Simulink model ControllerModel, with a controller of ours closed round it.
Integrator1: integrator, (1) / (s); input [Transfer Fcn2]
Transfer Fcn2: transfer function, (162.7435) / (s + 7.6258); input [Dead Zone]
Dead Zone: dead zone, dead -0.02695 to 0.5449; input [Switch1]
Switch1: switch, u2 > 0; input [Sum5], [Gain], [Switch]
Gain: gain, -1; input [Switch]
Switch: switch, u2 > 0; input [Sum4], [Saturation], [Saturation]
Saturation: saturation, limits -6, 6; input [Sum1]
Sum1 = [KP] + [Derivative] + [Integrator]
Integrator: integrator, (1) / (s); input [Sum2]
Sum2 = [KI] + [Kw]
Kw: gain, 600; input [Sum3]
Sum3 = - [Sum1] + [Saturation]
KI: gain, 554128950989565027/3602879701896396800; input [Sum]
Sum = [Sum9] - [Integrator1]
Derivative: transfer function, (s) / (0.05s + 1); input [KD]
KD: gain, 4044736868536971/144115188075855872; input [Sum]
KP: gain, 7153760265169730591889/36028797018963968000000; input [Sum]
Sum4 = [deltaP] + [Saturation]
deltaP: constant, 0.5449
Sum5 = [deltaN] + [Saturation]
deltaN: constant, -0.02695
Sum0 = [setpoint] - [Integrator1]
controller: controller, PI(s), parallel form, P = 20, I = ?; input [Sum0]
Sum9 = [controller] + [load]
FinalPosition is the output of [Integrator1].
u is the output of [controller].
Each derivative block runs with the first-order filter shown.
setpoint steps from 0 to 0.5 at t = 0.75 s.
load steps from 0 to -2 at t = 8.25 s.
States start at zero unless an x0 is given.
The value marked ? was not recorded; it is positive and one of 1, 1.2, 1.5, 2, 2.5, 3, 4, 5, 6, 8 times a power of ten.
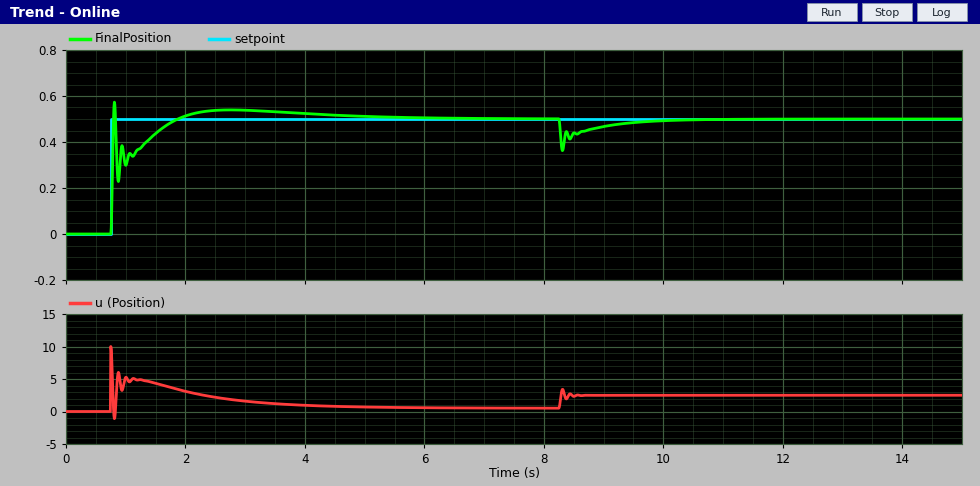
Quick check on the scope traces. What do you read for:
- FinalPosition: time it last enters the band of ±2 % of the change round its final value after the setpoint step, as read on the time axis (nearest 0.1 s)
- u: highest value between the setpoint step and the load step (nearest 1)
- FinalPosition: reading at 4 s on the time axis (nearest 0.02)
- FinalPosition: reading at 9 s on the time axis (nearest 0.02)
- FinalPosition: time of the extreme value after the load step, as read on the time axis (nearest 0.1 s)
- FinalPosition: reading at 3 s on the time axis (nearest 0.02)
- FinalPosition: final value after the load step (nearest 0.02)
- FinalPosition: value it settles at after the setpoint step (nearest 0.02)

5.2 s
10
0.52
0.46
8.3 s
0.54
0.50
0.50
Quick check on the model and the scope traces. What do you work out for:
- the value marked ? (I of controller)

30
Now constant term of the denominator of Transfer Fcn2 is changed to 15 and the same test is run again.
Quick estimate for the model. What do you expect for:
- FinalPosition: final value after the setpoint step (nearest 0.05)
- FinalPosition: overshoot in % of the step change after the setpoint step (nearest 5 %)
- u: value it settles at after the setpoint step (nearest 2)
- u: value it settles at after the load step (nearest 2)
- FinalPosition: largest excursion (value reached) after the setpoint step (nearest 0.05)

0.50
10 %
0
2
0.55
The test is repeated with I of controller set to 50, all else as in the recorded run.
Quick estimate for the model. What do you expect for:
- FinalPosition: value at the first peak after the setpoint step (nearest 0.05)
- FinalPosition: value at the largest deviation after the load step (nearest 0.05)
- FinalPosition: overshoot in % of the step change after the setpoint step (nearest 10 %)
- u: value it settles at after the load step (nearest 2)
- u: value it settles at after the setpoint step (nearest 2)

0.60
0.35
20 %
2
0
